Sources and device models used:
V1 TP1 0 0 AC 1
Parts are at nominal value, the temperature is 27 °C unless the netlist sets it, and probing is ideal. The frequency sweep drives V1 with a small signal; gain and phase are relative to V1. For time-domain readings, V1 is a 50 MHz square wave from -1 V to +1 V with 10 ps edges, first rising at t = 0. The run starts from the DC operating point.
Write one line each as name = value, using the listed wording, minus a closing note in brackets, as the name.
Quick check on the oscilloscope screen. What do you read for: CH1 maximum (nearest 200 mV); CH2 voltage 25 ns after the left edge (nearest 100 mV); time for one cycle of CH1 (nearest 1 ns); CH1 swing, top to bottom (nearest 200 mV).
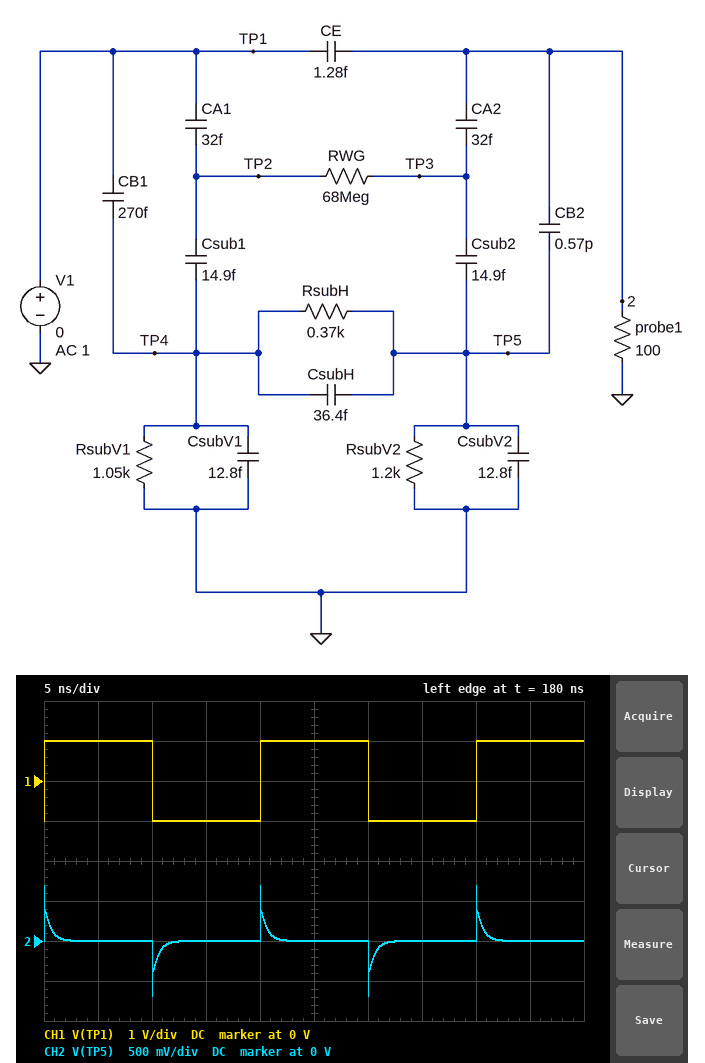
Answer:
CH1 maximum = 1.0 V
CH2 voltage 25 ns after the left edge = 0 V
time for one cycle of CH1 = 20 ns
CH1 swing, top to bottom = 2.0 V
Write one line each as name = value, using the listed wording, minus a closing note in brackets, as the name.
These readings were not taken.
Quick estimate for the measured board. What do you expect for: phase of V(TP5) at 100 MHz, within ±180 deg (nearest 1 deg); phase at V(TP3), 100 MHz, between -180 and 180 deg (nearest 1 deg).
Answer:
phase of V(TP5) at 100 MHz, within ±180 deg = 70 deg
phase at V(TP3), 100 MHz, between -180 and 180 deg = 75 deg
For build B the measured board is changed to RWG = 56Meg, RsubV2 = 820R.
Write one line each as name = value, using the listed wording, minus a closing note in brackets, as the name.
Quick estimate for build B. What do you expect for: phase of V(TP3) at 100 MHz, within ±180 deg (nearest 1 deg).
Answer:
phase of V(TP3) at 100 MHz, within ±180 deg = 78 deg
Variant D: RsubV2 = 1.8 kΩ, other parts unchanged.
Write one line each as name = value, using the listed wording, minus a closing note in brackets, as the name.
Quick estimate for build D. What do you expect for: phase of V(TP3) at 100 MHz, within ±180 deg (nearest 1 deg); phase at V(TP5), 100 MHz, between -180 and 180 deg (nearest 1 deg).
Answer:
phase of V(TP3) at 100 MHz, within ±180 deg = 71 deg
phase at V(TP5), 100 MHz, between -180 and 180 deg = 67 deg
